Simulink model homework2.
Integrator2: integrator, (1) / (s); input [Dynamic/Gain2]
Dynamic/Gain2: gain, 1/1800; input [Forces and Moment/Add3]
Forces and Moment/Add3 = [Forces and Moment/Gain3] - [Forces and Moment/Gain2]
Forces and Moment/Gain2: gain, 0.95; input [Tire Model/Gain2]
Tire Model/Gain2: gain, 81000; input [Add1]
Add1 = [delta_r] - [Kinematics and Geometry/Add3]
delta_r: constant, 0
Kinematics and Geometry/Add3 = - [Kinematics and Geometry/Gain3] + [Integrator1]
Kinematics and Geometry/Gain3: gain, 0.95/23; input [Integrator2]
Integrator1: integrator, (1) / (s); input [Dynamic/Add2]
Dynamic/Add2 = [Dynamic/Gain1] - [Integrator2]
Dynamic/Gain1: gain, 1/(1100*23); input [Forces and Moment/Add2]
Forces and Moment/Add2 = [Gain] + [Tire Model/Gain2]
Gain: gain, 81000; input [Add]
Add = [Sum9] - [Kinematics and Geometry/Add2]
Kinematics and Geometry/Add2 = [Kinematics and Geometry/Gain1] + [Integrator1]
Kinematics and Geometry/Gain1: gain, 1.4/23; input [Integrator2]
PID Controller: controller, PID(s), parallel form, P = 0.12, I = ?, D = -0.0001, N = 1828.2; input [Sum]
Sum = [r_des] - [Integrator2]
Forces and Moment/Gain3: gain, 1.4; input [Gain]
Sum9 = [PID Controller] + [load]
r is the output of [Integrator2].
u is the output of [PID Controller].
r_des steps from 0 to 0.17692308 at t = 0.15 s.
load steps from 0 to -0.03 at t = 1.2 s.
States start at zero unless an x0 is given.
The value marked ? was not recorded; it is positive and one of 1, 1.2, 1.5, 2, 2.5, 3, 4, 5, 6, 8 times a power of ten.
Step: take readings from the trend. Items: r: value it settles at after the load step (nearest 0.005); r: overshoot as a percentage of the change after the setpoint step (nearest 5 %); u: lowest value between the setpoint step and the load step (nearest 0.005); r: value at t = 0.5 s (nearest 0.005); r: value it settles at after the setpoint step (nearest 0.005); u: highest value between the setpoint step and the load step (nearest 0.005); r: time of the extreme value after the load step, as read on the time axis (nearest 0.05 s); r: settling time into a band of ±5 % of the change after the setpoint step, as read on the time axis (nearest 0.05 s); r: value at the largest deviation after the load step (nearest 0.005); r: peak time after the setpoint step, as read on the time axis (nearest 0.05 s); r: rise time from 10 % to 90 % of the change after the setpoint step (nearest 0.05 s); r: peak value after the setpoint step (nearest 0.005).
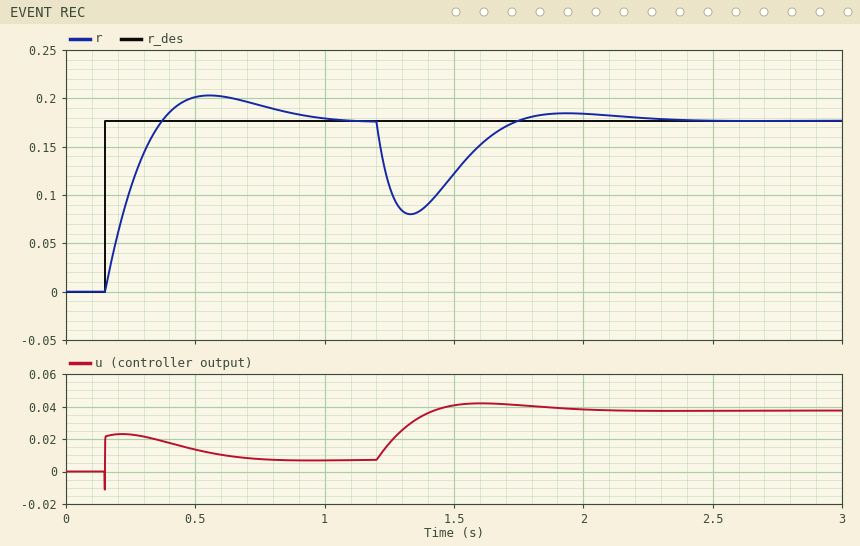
0.175
15 %
-0.010
0.200
0.175
0.025
1.35 s
0.85 s
0.080
0.55 s
0.15 s
0.205
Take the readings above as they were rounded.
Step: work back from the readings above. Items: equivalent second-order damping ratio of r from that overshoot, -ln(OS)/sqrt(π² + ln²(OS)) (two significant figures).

0.52
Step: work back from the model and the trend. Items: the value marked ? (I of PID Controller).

1.2
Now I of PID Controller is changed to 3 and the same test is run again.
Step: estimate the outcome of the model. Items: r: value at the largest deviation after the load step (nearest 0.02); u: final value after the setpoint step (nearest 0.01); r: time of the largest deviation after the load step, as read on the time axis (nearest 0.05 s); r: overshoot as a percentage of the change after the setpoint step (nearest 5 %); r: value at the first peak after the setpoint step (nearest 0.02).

0.10
0.01
1.30 s
25 %
0.22
